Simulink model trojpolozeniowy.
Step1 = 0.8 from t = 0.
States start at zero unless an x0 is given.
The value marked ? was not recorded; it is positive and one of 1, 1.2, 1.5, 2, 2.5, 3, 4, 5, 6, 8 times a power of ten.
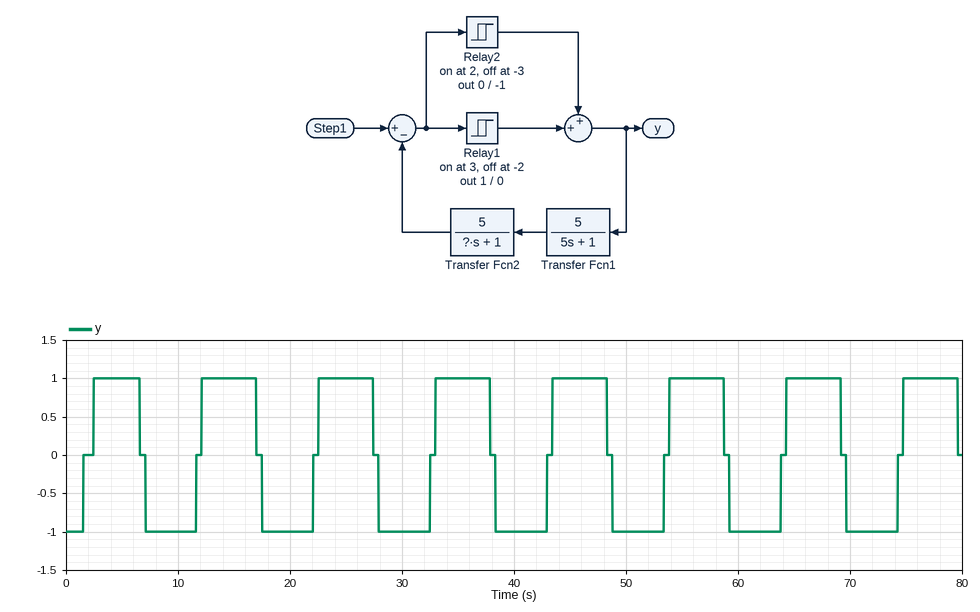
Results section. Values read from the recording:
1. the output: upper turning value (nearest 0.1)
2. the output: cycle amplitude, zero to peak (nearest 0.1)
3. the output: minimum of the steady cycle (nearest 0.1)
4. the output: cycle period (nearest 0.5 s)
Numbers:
1.0
1.0
-1.0
10.5 s
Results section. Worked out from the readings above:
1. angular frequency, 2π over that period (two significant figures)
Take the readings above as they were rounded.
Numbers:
0.60 rad/s
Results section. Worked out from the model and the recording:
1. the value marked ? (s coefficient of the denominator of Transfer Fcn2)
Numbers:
4
